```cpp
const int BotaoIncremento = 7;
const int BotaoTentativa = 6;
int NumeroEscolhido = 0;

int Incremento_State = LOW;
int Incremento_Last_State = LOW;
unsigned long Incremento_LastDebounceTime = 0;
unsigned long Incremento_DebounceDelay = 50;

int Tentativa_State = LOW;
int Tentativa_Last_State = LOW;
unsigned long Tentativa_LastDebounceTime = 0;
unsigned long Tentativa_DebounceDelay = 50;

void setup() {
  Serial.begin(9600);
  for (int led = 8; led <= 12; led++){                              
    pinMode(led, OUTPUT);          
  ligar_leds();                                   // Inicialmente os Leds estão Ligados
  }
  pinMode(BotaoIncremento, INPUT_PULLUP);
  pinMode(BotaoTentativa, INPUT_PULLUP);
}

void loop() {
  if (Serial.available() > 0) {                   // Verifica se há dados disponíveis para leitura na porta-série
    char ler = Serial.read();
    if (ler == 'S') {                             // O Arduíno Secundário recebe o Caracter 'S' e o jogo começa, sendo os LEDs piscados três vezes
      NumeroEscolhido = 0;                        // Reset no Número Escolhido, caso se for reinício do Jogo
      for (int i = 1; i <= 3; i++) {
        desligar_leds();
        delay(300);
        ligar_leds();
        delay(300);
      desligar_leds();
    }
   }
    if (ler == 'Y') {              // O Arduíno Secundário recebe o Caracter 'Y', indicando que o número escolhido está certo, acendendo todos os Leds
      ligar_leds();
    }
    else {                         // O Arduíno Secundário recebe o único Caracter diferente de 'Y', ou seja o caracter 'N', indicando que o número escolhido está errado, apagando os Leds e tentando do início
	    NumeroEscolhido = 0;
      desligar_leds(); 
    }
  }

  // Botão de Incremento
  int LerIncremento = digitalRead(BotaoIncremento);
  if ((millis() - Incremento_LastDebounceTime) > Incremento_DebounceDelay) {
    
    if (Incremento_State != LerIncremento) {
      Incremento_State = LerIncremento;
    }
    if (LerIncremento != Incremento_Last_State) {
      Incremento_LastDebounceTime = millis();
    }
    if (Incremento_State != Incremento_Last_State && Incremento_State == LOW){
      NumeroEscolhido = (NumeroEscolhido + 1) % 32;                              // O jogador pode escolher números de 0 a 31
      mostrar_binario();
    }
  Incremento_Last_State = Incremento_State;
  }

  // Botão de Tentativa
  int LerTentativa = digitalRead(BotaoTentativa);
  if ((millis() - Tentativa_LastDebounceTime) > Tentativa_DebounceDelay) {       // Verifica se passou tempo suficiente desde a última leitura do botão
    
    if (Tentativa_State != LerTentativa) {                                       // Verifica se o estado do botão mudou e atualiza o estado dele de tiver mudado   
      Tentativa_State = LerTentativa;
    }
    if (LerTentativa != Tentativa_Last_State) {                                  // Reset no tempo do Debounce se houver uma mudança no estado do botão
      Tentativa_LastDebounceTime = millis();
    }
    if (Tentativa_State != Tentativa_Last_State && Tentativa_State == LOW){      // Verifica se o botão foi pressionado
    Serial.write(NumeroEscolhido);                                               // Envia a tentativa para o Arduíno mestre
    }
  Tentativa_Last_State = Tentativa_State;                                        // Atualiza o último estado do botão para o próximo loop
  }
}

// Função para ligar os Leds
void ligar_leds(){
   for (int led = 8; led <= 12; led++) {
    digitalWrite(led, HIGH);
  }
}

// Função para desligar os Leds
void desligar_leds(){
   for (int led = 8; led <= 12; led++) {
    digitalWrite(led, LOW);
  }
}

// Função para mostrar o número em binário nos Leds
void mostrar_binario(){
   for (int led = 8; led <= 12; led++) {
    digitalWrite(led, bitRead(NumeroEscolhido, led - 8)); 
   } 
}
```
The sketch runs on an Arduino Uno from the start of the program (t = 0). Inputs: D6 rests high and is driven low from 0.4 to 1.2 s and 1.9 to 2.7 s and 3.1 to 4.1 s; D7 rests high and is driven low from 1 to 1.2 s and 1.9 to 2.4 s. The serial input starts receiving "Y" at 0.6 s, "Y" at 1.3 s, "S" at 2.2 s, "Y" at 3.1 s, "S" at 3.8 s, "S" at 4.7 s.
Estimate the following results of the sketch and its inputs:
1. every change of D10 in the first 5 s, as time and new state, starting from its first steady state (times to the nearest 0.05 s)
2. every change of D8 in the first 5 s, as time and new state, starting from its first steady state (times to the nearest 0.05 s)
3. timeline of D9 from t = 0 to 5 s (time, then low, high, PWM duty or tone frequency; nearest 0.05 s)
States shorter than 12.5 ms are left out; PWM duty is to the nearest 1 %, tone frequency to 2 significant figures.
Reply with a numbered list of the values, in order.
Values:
1. 0 s high; 1 s low; 1.3 s high; 1.9 s low; 2.5 s high; 2.8 s low; 3.1 s high; 3.4 s low; 3.7 s high; 4 s low; 4.3 s high; 4.6 s low; 4.9 s high
2. 0 s high; 1.9 s low; 2.5 s high; 2.8 s low; 3.1 s high; 3.4 s low; 3.7 s high; 4 s low; 4.3 s high; 4.6 s low; 4.9 s high
3. 0 s high; 1 s low; 1.3 s high; 2.2 s low; 2.5 s high; 2.8 s low; 3.1 s high; 3.4 s low; 3.7 s high; 4 s low; 4.3 s high; 4.6 s low; 4.9 s high
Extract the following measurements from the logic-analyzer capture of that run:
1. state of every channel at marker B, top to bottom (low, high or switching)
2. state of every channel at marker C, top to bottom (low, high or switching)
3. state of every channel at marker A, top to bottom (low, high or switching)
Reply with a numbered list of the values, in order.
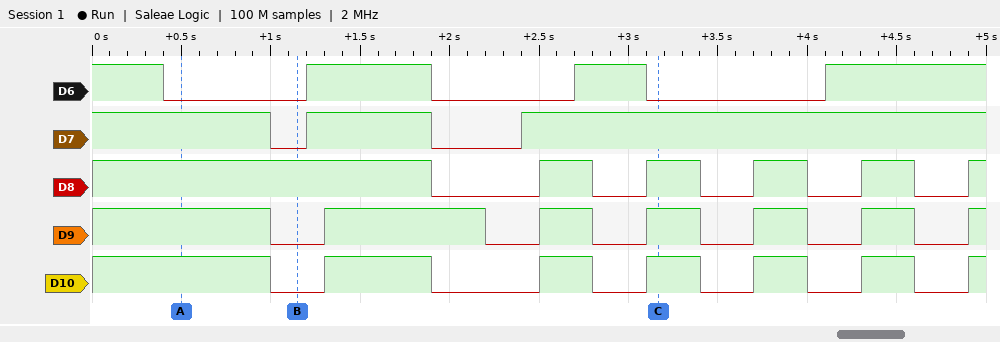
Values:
1. D6 low, D7 low, D8 high, D9 low, D10 low
2. D6 low, D7 high, D8 high, D9 high, D10 high
3. D6 low, D7 high, D8 high, D9 high, D10 high
